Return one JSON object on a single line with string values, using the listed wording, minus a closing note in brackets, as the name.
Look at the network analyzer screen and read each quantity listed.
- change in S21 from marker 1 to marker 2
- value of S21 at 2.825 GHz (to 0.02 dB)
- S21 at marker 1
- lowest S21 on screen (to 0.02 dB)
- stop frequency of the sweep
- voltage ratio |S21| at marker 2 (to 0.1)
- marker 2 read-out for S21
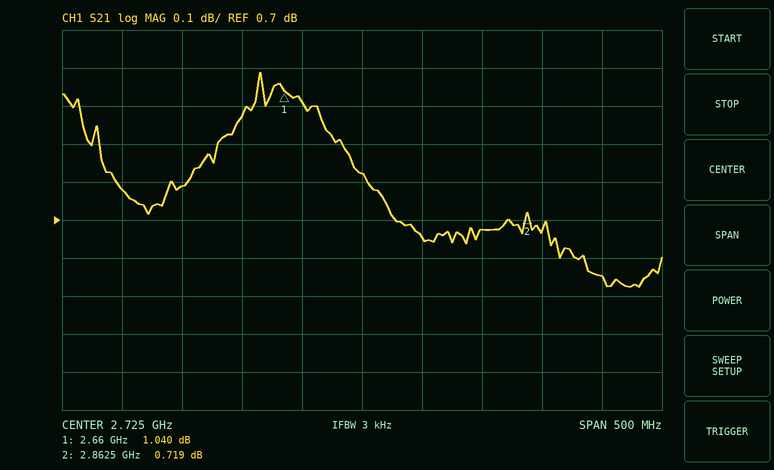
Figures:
{"change in S21 from marker 1 to marker 2": "-0.321 dB", "value of S21 at 2.825 GHz": "0.68 dB", "S21 at marker 1": "1.040 dB", "lowest S21 on screen": "0.52 dB", "stop frequency of the sweep": "2.975 GHz", "voltage ratio |S21| at marker 2": "1.1", "marker 2 read-out for S21": "0.719 dB"}
